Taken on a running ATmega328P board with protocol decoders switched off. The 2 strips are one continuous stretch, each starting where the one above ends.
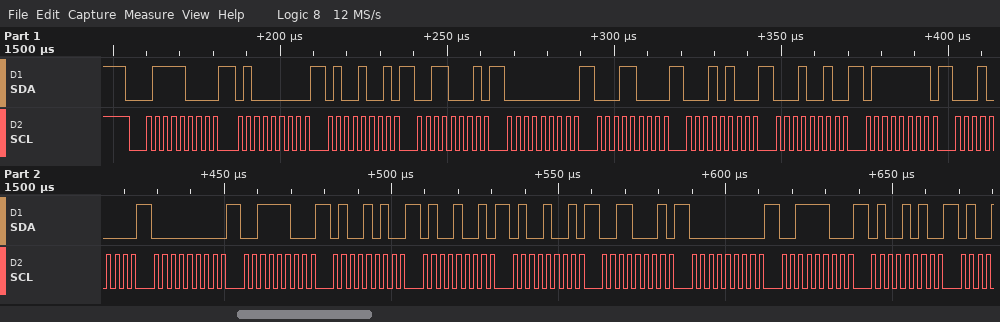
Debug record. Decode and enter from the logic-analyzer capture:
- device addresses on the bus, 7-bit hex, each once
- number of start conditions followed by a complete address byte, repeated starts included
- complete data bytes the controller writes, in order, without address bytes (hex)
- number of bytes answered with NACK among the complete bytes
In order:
0x3C
1
40 49 31 00 18 14 12 7F 10 00 3C 4A 49 49 31 00 3C 4A
0
